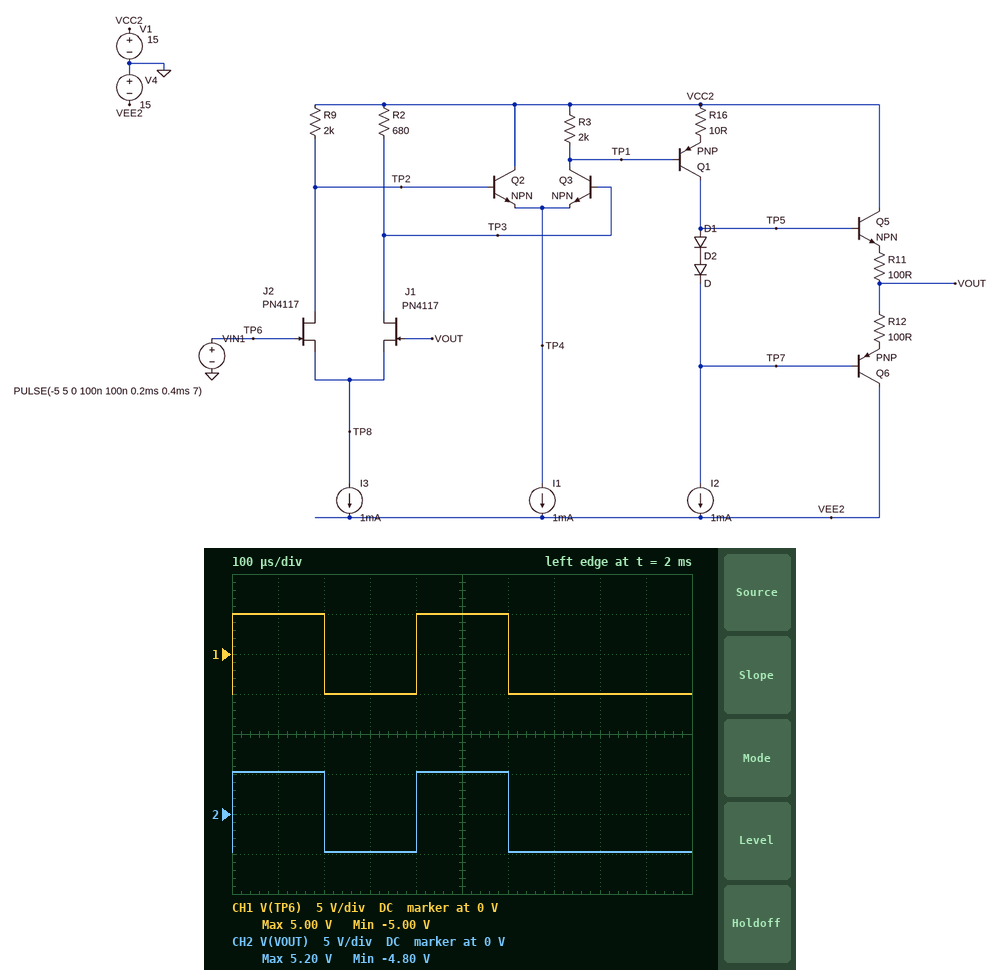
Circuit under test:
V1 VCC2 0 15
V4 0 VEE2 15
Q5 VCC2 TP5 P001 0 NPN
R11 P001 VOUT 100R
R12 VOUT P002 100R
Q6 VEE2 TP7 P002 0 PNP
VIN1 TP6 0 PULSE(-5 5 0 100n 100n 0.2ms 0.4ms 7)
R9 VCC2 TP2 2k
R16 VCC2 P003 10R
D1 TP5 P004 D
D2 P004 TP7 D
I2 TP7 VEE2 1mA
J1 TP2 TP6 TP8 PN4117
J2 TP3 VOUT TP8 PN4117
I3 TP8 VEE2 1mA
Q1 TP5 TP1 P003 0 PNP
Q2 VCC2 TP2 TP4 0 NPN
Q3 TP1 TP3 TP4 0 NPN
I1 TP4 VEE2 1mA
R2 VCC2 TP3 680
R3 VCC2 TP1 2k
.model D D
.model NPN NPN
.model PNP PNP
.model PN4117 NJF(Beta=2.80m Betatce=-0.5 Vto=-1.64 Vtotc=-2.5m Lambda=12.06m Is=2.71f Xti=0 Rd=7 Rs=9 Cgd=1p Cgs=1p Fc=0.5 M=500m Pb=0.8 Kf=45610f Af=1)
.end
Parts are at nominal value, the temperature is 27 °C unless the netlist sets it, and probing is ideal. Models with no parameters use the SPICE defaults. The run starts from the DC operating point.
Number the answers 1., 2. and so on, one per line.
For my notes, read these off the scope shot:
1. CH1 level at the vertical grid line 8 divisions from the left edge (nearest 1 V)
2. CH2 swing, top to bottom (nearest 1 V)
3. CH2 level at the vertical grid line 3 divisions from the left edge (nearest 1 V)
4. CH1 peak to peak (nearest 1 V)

1. -5 V
2. 10 V
3. -5 V
4. 10 V
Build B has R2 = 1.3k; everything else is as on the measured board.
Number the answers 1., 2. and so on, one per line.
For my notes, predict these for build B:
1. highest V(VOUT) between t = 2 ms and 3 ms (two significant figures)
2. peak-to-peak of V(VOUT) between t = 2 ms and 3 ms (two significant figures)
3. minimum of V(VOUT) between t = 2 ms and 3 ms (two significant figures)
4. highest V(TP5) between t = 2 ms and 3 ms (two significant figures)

1. 5.1 V
2. 10 V
3. -4.9 V
4. 5.8 V
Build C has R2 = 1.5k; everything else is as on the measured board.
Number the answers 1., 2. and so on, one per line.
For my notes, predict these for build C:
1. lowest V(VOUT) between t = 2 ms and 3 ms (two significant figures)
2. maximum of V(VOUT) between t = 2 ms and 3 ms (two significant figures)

1. -4.9 V
2. 5.1 V
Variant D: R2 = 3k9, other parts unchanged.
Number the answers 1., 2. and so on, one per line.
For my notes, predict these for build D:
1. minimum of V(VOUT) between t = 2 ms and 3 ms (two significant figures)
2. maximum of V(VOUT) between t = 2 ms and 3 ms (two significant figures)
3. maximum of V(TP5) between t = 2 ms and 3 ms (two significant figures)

1. -5.1 V
2. 4.9 V
3. 5.6 V
